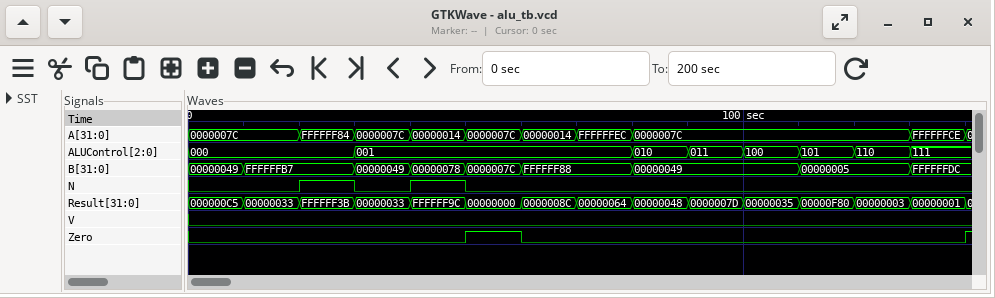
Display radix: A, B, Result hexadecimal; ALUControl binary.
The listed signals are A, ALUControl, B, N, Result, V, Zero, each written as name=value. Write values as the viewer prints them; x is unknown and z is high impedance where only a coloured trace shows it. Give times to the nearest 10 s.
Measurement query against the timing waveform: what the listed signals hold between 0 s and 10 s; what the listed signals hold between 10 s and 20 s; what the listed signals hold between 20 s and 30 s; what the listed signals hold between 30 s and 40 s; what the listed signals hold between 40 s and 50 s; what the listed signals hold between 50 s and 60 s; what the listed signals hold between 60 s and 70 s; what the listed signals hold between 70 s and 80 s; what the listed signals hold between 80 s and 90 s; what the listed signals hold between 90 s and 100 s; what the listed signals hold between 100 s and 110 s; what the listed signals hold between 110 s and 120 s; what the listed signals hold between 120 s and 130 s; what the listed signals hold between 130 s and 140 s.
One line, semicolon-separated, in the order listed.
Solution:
A=0000007C, ALUControl=000, B=00000049, N=0, Result=000000C5, V=0, Zero=0; A=0000007C, ALUControl=000, B=FFFFFFB7, N=0, Result=00000033, V=0, Zero=0; A=FFFFFF84, ALUControl=000, B=FFFFFFB7, N=1, Result=FFFFFF3B, V=0, Zero=0; A=0000007C, ALUControl=001, B=00000049, N=0, Result=00000033, V=0, Zero=0; A=00000014, ALUControl=001, B=00000078, N=1, Result=FFFFFF9C, V=0, Zero=0; A=0000007C, ALUControl=001, B=0000007C, N=0, Result=00000000, V=0, Zero=1; A=00000014, ALUControl=001, B=FFFFFF88, N=0, Result=0000008C, V=0, Zero=0; A=FFFFFFEC, ALUControl=001, B=FFFFFF88, N=0, Result=00000064, V=0, Zero=0; A=0000007C, ALUControl=010, B=00000049, N=0, Result=00000048, V=0, Zero=0; A=0000007C, ALUControl=011, B=00000049, N=0, Result=0000007D, V=0, Zero=0; A=0000007C, ALUControl=100, B=00000049, N=0, Result=00000035, V=0, Zero=0; A=0000007C, ALUControl=101, B=00000005, N=0, Result=00000F80, V=0, Zero=0; A=0000007C, ALUControl=110, B=00000005, N=0, Result=00000003, V=0, Zero=0; A=FFFFFFCE, ALUControl=111, B=FFFFFFDC, N=0, Result=00000001, V=0, Zero=0
